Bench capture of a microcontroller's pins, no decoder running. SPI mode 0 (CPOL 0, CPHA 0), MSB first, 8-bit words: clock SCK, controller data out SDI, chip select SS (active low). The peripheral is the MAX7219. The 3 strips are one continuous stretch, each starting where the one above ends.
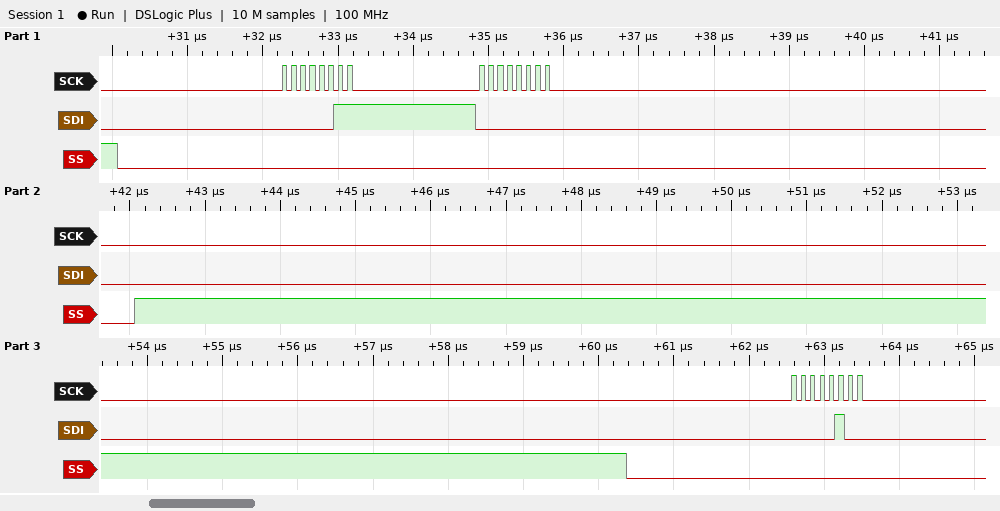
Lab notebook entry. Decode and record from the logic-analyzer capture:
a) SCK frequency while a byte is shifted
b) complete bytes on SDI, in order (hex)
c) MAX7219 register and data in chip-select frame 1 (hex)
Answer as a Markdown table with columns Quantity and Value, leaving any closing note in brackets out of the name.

| Quantity | Value |
|---|---|
| SCK frequency while a byte is shifted | 8 MHz |
| complete bytes on SDI, in order | 03 00 04 |
| MAX7219 register and data in chip-select frame 1 | register 0x3, data 0x00 |
